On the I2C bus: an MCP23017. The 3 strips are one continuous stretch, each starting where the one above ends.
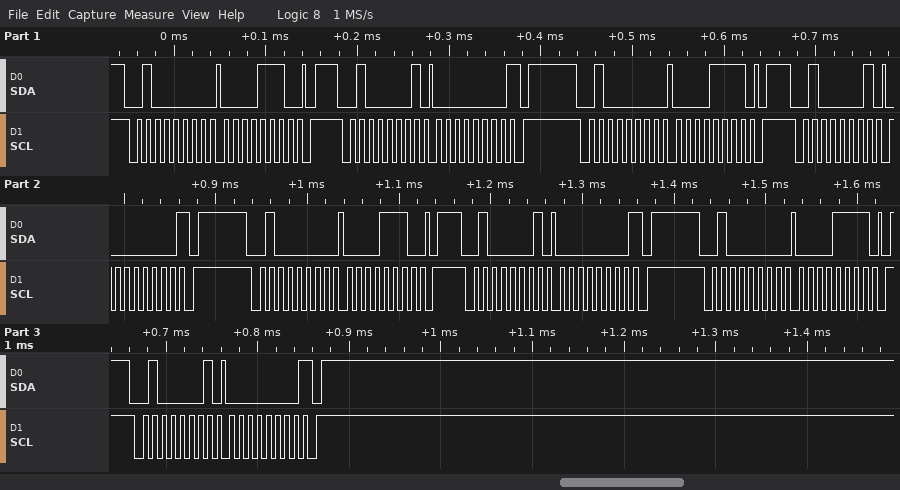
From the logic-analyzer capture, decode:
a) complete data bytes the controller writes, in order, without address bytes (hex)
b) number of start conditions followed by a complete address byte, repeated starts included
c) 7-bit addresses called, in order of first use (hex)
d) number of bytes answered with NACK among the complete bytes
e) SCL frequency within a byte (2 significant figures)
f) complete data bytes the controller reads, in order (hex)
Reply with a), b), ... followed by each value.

a) 0E 0F 0E 0F
b) 8
c) 0x20
d) 4
e) 100 kHz
f) 00 00 00 00
